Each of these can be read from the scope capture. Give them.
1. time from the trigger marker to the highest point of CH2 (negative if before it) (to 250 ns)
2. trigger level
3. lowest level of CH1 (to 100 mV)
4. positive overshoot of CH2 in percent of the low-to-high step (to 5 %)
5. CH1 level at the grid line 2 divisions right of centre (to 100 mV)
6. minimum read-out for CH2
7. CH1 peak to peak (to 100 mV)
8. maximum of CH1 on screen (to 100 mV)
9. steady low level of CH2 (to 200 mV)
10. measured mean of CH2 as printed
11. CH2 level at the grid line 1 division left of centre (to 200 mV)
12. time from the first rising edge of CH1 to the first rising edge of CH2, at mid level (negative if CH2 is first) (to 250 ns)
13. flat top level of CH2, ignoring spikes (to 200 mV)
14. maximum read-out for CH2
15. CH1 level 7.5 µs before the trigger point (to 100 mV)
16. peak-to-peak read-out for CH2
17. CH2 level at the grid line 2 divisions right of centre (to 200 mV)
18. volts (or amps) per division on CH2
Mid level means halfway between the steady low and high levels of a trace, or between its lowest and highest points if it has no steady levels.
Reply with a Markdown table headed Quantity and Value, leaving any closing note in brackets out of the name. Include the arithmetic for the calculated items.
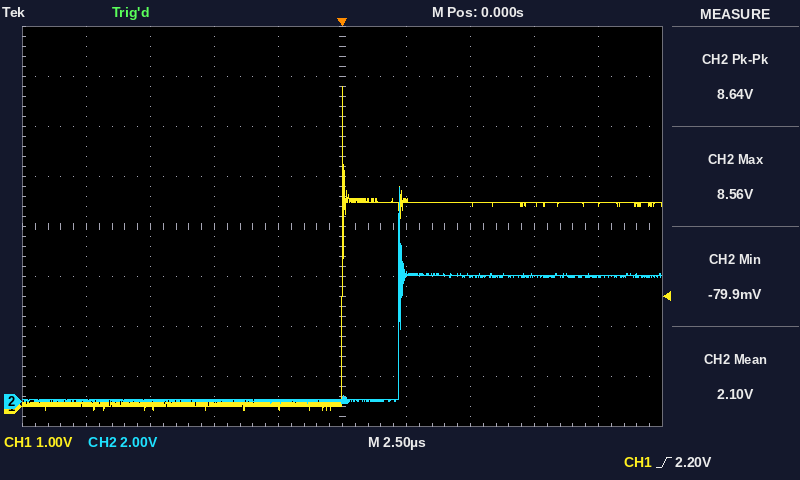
| Quantity | Value |
|---|---|
| time from the trigger marker to the highest point of CH2 (negative if before it) | +2.25 µs |
| trigger level | 2.20 V |
| lowest level of CH1 | -100 mV |
| positive overshoot of CH2 in percent of the low-to-high step | 70 % |
| CH1 level at the grid line 2 divisions right of centre | 4.0 V |
| minimum read-out for CH2 | -79.9 mV |
| CH1 peak to peak | 6.4 V − (-100 mV) = 6.5 V |
| maximum of CH1 on screen | 6.4 V |
| steady low level of CH2 | 0.0 V |
| measured mean of CH2 as printed | 2.10 V |
| CH2 level at the grid line 1 division left of centre | 0.0 V |
| time from the first rising edge of CH1 to the first rising edge of CH2, at mid level (negative if CH2 is first) | +2.25 µs |
| flat top level of CH2, ignoring spikes | 5.0 V |
| maximum read-out for CH2 | 8.56 V |
| CH1 level 7.5 µs before the trigger point | 0.0 V |
| peak-to-peak read-out for CH2 | 8.64 V |
| CH2 level at the grid line 2 divisions right of centre | 5.0 V |
| volts (or amps) per division on CH2 | 2 V |
